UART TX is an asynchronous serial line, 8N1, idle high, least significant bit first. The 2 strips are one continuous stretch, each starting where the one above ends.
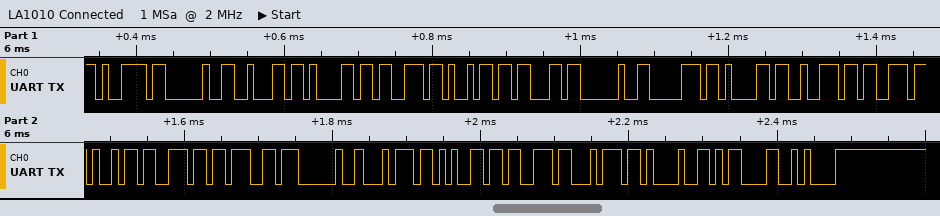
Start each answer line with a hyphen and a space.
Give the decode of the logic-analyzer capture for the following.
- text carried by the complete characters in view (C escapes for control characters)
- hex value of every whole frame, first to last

- "y basic parsing test!\r\n"
- 0x79 0x20 0x62 0x61 0x73 0x69 0x63 0x20 0x70 0x61 0x72 0x73 0x69 0x6E 0x67 0x20 0x74 0x65 0x73 0x74 0x21 0x0D 0x0A
